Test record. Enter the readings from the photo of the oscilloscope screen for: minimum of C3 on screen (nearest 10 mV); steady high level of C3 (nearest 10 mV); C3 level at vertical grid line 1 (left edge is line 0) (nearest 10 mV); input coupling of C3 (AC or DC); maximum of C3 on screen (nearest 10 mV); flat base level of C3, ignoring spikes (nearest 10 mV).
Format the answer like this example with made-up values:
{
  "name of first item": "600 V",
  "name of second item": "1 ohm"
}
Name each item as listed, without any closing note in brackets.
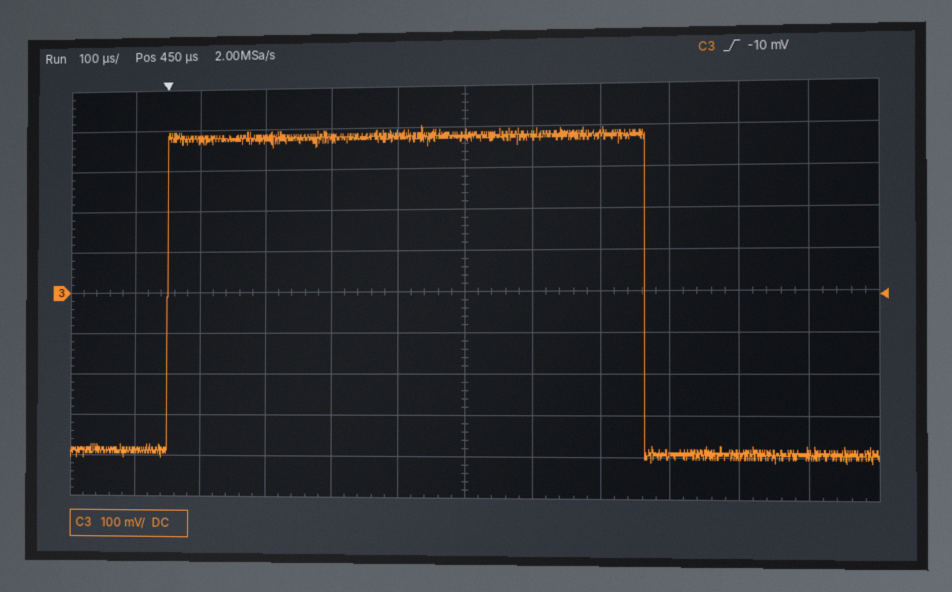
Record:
{
  "minimum of C3 on screen": "-410 mV",
  "steady high level of C3": "380 mV",
  "C3 level at vertical grid line 1 (left edge is line 0)": "-390 mV",
  "input coupling of C3": "DC",
  "maximum of C3 on screen": "400 mV",
  "flat base level of C3, ignoring spikes": "-390 mV"
}
